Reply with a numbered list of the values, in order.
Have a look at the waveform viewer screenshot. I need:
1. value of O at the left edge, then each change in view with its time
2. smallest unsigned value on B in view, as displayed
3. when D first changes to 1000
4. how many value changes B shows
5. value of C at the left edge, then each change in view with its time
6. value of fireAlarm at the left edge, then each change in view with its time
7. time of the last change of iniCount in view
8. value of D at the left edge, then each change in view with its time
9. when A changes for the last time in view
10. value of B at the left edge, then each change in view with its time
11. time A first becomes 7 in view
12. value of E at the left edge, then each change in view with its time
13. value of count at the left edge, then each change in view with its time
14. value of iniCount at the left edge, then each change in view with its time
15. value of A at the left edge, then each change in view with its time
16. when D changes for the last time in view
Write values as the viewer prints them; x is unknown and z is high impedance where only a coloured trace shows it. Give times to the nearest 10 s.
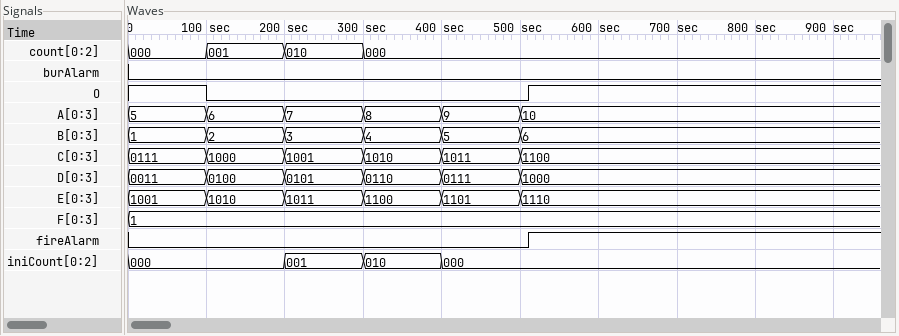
1. 1, 0 at 100 s, 1 at 510 s
2. 1
3. 500 s
4. 5
5. 0111, 1000 at 100 s, 1001 at 200 s, 1010 at 300 s, 1011 at 400 s, 1100 at 500 s
6. 0, 1 at 510 s
7. 400 s
8. 0011, 0100 at 100 s, 0101 at 200 s, 0110 at 300 s, 0111 at 400 s, 1000 at 500 s
9. 500 s
10. 1, 2 at 100 s, 3 at 200 s, 4 at 300 s, 5 at 400 s, 6 at 500 s
11. 200 s
12. 1001, 1010 at 100 s, 1011 at 200 s, 1100 at 300 s, 1101 at 400 s, 1110 at 500 s
13. 000, 001 at 100 s, 010 at 200 s, 000 at 300 s
14. 000, 001 at 200 s, 010 at 300 s, 000 at 400 s
15. 5, 6 at 100 s, 7 at 200 s, 8 at 300 s, 9 at 400 s, 10 at 500 s
16. 500 s
